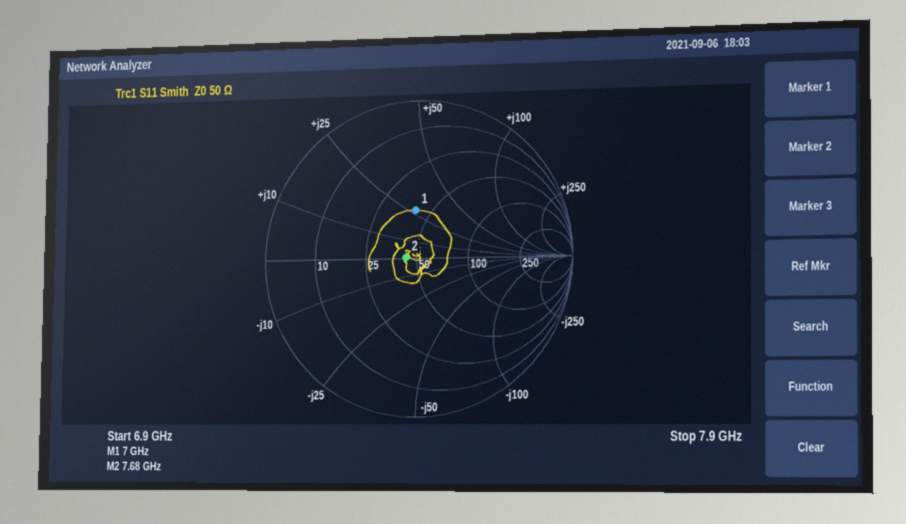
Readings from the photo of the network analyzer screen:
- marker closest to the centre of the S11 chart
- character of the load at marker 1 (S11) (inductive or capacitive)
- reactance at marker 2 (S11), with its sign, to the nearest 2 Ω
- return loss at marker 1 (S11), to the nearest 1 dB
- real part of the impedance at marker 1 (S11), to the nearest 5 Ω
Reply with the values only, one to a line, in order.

marker 2
inductive
0 Ω
10 dB
40 Ω
